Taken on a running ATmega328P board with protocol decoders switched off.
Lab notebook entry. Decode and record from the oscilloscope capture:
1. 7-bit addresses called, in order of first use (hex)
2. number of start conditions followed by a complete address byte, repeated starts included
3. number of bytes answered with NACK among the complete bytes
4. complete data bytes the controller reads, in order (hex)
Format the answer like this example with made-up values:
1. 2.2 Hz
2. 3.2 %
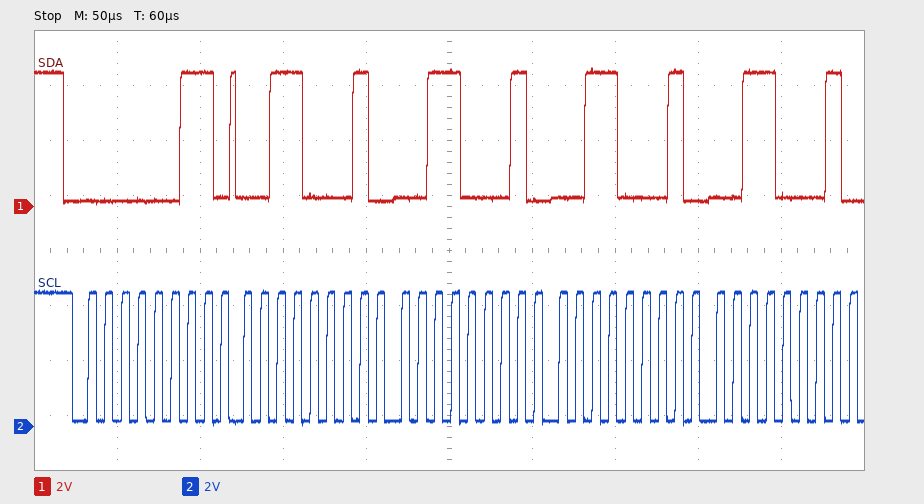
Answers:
1. 0x01
2. 1
3. 0
4. 31 31 31 31
